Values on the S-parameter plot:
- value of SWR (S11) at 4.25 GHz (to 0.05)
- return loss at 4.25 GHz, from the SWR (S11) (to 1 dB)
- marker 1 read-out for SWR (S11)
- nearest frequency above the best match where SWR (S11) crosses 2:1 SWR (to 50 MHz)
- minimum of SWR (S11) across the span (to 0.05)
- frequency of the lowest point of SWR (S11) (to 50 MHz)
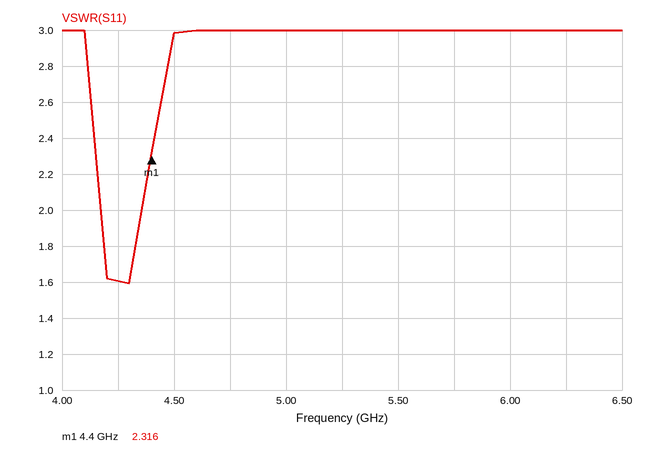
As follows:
1.60
13 dB
2.316
4.35 GHz
1.60
4.30 GHz
